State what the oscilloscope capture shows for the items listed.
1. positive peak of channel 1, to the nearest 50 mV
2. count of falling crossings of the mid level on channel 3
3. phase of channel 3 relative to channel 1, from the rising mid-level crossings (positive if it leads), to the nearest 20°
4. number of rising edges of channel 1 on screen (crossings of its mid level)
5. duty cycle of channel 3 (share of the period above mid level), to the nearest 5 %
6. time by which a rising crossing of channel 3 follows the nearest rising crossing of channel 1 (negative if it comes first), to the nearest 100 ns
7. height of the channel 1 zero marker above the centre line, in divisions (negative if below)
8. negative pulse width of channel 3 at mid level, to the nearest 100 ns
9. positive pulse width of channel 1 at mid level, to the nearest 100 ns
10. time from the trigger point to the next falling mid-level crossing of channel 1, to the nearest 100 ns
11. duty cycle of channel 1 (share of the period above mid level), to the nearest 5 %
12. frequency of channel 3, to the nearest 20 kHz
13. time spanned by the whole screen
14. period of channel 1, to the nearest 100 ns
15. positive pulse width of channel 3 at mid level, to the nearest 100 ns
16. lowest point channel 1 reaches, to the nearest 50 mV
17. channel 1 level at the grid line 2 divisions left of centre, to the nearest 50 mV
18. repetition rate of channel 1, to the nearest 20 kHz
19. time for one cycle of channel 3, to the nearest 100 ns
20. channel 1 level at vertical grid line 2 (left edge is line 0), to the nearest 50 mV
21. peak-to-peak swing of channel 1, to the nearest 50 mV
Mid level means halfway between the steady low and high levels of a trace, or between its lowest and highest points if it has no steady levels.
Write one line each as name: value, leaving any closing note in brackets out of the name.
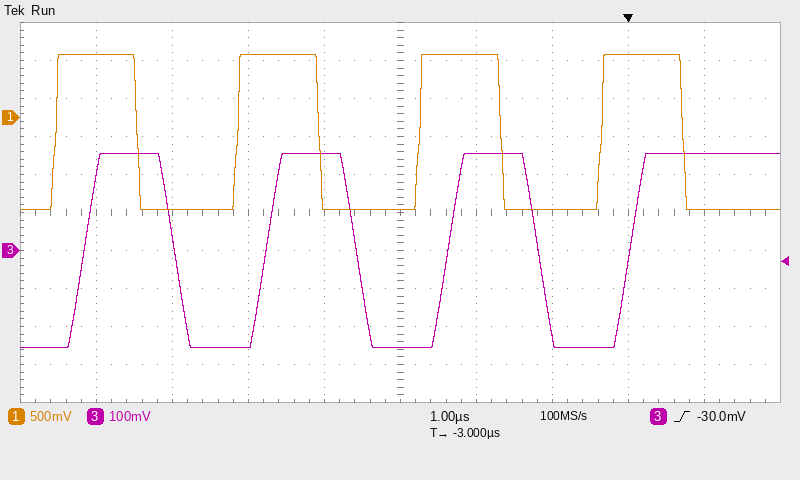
positive peak of channel 1, to the nearest 50 mV: 850 mV
count of falling crossings of the mid level on channel 3: 3
phase of channel 3 relative to channel 1, from the rising mid-level crossings (positive if it leads), to the nearest 20°: -60°
number of rising edges of channel 1 on screen: 4
duty cycle of channel 3 (share of the period above mid level), to the nearest 5 %: 50 %
time by which a rising crossing of channel 3 follows the nearest rising crossing of channel 1 (negative if it comes first), to the nearest 100 ns: +400 ns
height of the channel 1 zero marker above the centre line, in divisions: +2.5 div
negative pulse width of channel 3 at mid level, to the nearest 100 ns: 1.2 µs
positive pulse width of channel 1 at mid level, to the nearest 100 ns: 1.1 µs
time from the trigger point to the next falling mid-level crossing of channel 1, to the nearest 100 ns: 700 ns
duty cycle of channel 1 (share of the period above mid level), to the nearest 5 %: 45 %
frequency of channel 3, to the nearest 20 kHz: 420 kHz
time spanned by the whole screen: 10 µs
period of channel 1, to the nearest 100 ns: 2.4 µs
positive pulse width of channel 3 at mid level, to the nearest 100 ns: 1.2 µs
lowest point channel 1 reaches, to the nearest 50 mV: -1.20 V
channel 1 level at the grid line 2 divisions left of centre, to the nearest 50 mV: 850 mV
repetition rate of channel 1, to the nearest 20 kHz: 420 kHz
time for one cycle of channel 3, to the nearest 100 ns: 2.4 µs
channel 1 level at vertical grid line 2 (left edge is line 0), to the nearest 50 mV: -1.20 V
peak-to-peak swing of channel 1, to the nearest 50 mV: 2.05 V
